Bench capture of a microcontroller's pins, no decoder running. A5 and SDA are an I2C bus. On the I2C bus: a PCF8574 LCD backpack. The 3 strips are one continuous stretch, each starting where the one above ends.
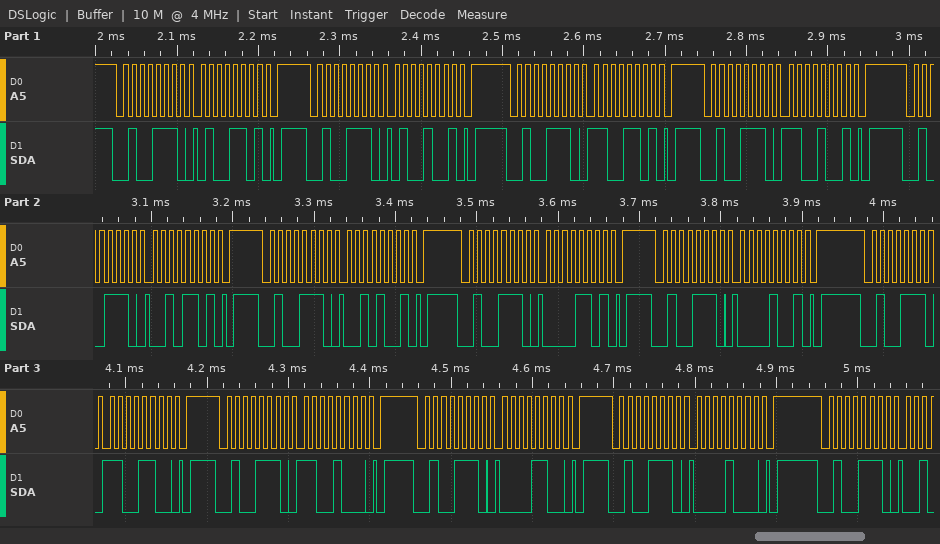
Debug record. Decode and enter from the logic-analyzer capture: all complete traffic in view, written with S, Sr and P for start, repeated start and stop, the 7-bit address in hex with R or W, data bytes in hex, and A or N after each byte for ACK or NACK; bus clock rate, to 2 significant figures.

S 27W A 4D A P S 27W A 49 A P S 27W A CD A P S 27W A C9 A P S 27W A 2D A P S 27W A 29 A P S 27W A 0D A P S 27W A 09 A P S 27W A CC A P S 27W A C8 A P S 27W A 0C A P S 27W A 08 A P S 27W A
100 kHz
